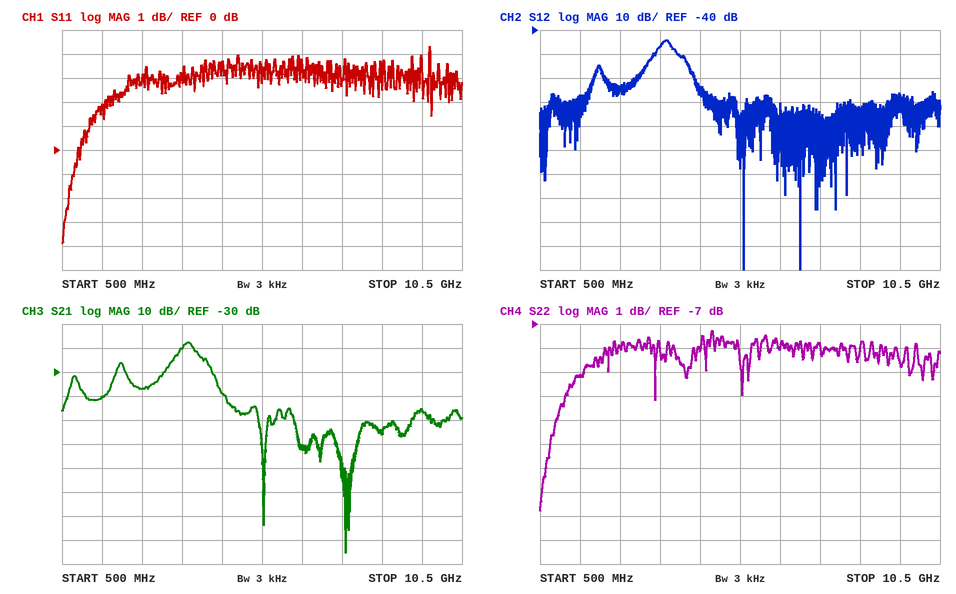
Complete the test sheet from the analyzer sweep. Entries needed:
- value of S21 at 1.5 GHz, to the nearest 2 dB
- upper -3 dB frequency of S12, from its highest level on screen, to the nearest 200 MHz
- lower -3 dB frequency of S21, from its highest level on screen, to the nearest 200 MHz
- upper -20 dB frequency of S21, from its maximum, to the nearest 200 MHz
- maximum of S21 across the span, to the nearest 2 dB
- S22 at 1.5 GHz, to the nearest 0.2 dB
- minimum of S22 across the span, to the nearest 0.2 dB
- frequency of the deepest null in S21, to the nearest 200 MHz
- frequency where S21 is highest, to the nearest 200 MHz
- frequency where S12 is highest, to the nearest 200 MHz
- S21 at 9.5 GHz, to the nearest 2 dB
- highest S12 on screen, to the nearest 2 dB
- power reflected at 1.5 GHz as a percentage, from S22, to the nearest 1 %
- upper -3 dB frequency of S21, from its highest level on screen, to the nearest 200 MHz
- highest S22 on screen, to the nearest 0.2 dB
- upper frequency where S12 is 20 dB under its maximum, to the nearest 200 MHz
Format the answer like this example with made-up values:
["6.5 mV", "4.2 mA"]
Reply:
["-40 dB", "3.8 GHz", "3.4 GHz", "4.4 GHz", "-18 dB", "-9.2 dB", "-14.8 dB", "7.6 GHz", "3.6 GHz", "3.6 GHz", "-46 dB", "-44 dB", "12 %", "3.8 GHz", "-7.2 dB", "4.4 GHz"]
